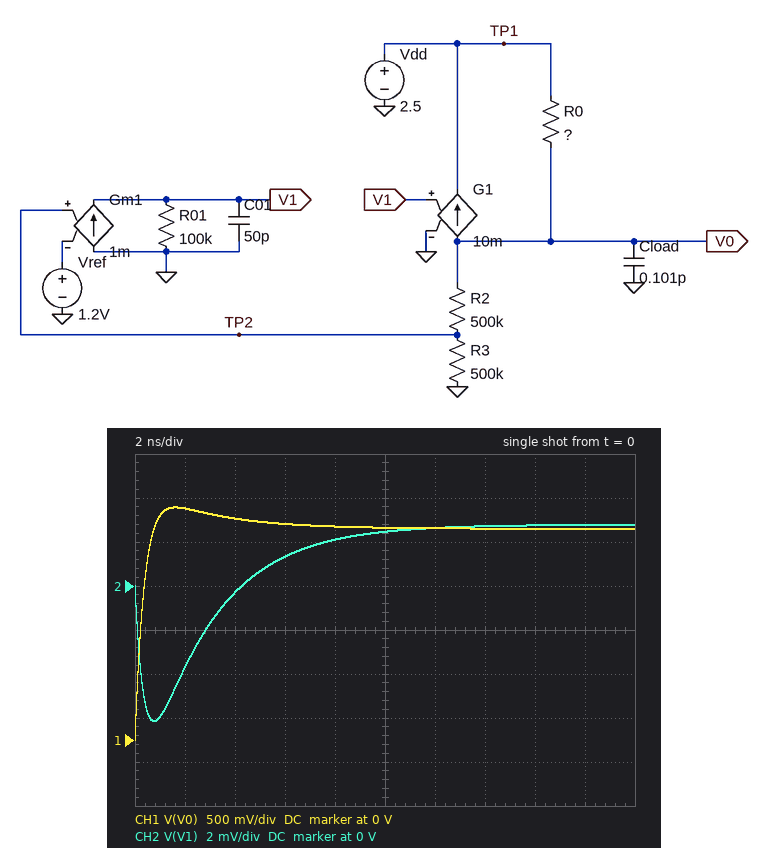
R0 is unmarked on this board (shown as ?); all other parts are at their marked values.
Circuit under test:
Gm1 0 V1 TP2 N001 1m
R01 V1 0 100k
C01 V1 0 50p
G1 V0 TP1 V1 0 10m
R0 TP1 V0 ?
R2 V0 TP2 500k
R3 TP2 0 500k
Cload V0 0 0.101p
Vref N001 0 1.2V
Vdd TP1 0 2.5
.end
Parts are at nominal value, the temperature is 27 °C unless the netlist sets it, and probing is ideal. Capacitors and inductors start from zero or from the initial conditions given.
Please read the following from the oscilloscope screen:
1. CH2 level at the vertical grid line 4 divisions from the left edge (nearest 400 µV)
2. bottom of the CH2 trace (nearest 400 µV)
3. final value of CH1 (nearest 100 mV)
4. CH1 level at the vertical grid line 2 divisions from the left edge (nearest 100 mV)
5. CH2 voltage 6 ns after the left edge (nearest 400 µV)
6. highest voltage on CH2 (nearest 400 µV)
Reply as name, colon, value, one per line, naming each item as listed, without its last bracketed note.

CH2 level at the vertical grid line 4 divisions from the left edge: 2.0 mV
bottom of the CH2 trace: -6.0 mV
final value of CH1: 2.4 V
CH1 level at the vertical grid line 2 divisions from the left edge: 2.5 V
CH2 voltage 6 ns after the left edge: 1.2 mV
highest voltage on CH2: 2.8 mV
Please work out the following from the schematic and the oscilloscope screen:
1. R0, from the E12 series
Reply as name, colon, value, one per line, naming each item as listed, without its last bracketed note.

R0, from the E12 series: 3.3 kΩ
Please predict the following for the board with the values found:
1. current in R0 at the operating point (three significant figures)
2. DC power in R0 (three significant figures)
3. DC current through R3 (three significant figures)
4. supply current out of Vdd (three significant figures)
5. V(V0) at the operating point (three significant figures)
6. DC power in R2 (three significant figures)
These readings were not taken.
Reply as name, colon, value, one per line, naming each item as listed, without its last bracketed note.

current in R0 at the operating point: 30.3 µA
DC power in R0: 3.03 µW
DC current through R3: 2.40 µA
supply current out of Vdd: 2.40 µA
V(V0) at the operating point: 2.40 V
DC power in R2: 2.88 µW
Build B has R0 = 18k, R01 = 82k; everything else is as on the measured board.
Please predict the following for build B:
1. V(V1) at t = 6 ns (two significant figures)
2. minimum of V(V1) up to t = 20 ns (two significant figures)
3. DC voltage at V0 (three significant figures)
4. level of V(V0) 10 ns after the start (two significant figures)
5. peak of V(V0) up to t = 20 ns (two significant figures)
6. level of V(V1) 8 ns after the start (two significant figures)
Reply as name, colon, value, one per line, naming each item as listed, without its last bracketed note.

V(V1) at t = 6 ns: 2.7 mV
minimum of V(V1) up to t = 20 ns: -16 mV
DC voltage at V0: 2.40 V
level of V(V0) 10 ns after the start: 2.5 V
peak of V(V0) up to t = 20 ns: 3.5 V
level of V(V1) 8 ns after the start: -2.3 mV
